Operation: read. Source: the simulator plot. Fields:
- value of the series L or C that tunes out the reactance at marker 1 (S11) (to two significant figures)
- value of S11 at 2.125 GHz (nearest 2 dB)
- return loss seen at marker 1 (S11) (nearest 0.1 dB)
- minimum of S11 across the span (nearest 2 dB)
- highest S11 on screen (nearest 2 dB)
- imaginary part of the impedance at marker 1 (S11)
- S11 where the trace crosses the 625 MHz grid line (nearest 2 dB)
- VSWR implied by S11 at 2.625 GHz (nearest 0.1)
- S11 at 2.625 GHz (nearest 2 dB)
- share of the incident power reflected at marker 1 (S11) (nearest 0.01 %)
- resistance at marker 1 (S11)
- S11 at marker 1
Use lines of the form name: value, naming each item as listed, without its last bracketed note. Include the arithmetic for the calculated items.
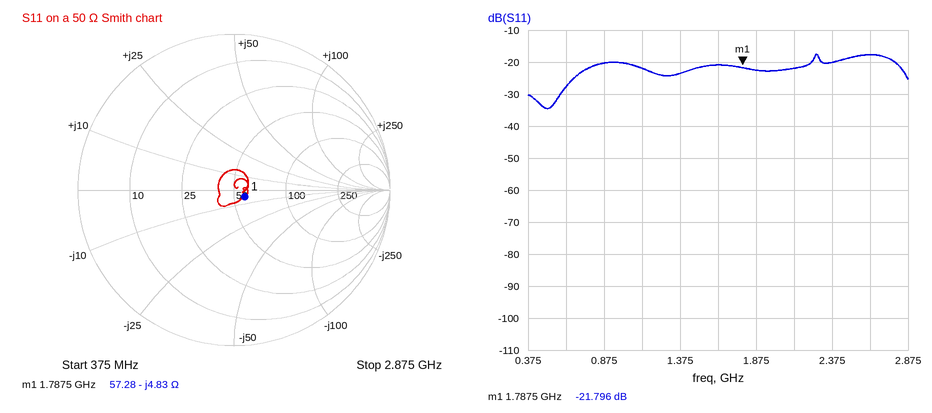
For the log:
value of the series L or C that tunes out the reactance at marker 1 (S11): L = 4.83 Ω/(2π × 1.7875 GHz) ≈ 430 pH
value of S11 at 2.125 GHz: -22 dB
return loss seen at marker 1 (S11): 21.8 dB
minimum of S11 across the span: -34 dB
highest S11 on screen: -18 dB
imaginary part of the impedance at marker 1: -4.83 Ω
S11 where the trace crosses the 625 MHz grid line: -28 dB
VSWR implied by S11 at 2.625 GHz: |Γ| = 10^(-18/20) = 0.1259; VSWR = (1 + 0.1259)/(1 − 0.1259) ≈ 1.3
S11 at 2.625 GHz: -18 dB
share of the incident power reflected at marker 1 (S11): 10^(-21.796/10) ≈ 0.66 %
resistance at marker 1: 57.28 Ω
S11 at marker 1: -21.796 dB
